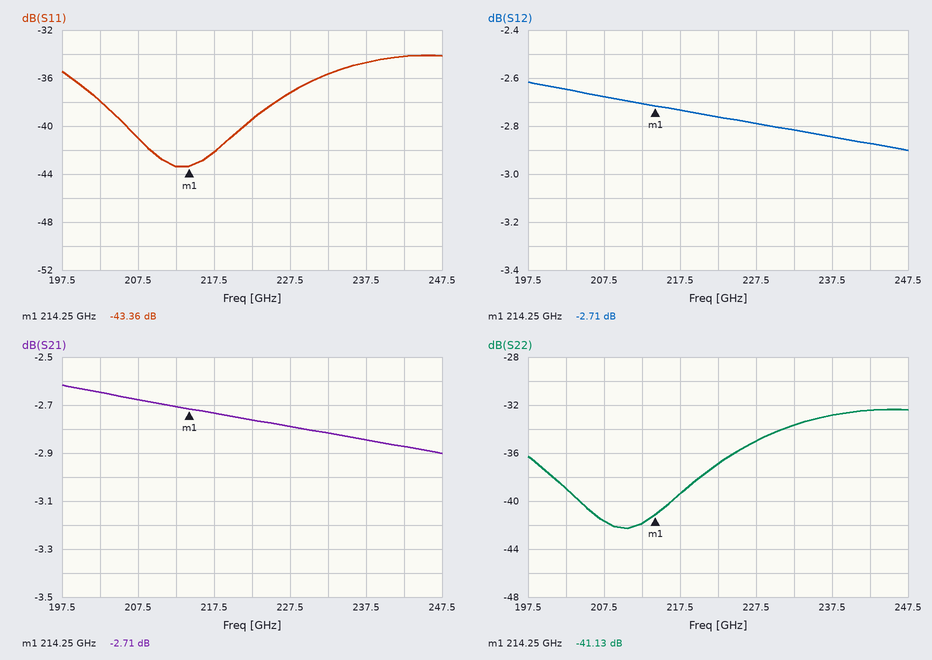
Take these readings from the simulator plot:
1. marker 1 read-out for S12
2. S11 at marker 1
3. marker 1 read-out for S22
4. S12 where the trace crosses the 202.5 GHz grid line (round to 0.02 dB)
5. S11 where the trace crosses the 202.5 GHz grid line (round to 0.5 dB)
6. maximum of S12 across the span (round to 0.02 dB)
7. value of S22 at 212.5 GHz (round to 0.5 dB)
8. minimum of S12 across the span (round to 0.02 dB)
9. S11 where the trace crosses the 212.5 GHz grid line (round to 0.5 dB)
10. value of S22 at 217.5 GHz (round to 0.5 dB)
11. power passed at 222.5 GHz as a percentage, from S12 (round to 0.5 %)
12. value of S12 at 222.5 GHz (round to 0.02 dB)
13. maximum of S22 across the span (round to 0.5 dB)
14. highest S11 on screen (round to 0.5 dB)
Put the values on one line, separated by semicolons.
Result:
-2.71 dB; -43.36 dB; -41.13 dB; -2.64 dB; -38.0 dB; -2.62 dB; -42.0 dB; -2.90 dB; -43.5 dB; -39.5 dB; 53.0 %; -2.76 dB; -32.5 dB; -34.0 dB
